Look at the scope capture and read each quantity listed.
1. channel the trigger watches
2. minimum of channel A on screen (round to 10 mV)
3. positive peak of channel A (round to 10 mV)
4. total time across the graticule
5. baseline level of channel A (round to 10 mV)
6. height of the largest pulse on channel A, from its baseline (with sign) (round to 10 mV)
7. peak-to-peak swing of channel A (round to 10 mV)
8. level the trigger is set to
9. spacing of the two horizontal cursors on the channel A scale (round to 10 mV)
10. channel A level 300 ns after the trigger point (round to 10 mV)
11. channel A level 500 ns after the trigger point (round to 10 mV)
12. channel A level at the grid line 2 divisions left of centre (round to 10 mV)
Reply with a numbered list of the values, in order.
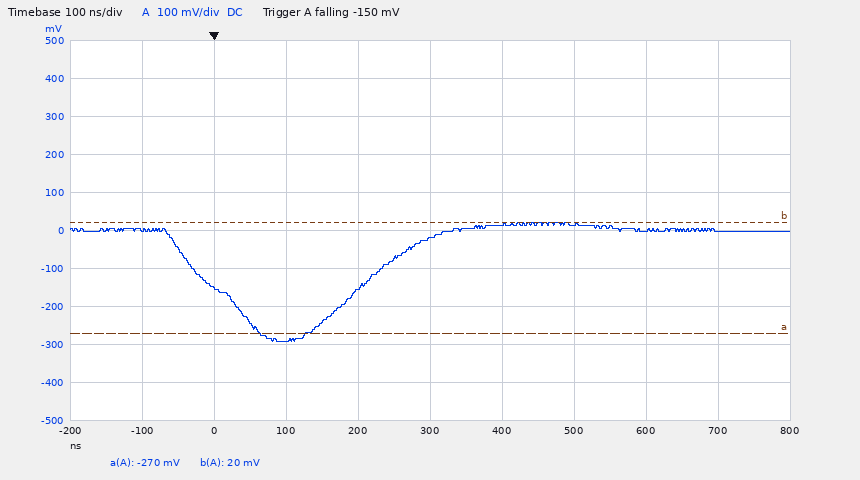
1. channel A
2. -290 mV
3. 20 mV
4. 1 µs
5. 0 mV
6. -290 mV
7. 310 mV
8. -150 mV
9. 290 mV
10. -20 mV
11. 20 mV
12. -290 mV
